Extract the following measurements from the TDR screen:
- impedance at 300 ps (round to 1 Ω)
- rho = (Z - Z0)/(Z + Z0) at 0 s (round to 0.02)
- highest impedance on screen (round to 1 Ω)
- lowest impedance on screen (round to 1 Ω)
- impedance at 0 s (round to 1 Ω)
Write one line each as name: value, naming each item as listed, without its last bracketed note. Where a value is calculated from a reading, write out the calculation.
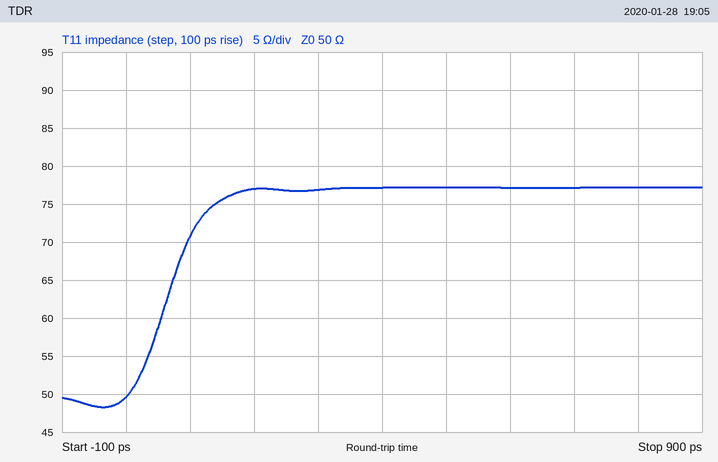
impedance at 300 ps: 77 Ω
rho = (Z - Z0)/(Z + Z0) at 0 s: (50 − 50)/(50 + 50) ≈ 0.00
highest impedance on screen: 77 Ω
lowest impedance on screen: 48 Ω
impedance at 0 s: 50 Ω
